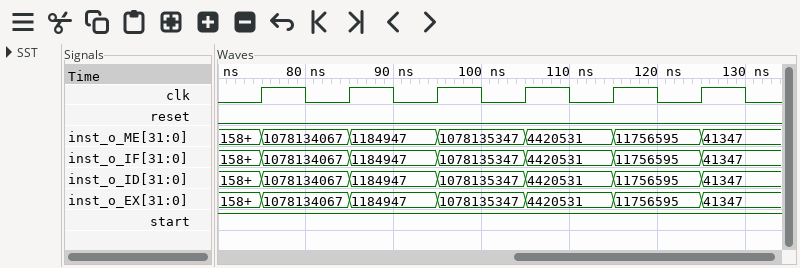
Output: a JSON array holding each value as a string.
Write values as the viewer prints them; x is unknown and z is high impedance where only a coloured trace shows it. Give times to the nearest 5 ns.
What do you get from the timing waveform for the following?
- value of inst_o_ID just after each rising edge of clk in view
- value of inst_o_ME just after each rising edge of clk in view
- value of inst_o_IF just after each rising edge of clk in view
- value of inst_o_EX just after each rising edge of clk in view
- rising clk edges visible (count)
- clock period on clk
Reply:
["1078134067, 1184947, 1078135347, 4420531, 11756595, 41347", "1078134067, 1184947, 1078135347, 4420531, 11756595, 41347", "1078134067, 1184947, 1078135347, 4420531, 11756595, 41347", "1078134067, 1184947, 1078135347, 4420531, 11756595, 41347", "6", "10 ns"]
